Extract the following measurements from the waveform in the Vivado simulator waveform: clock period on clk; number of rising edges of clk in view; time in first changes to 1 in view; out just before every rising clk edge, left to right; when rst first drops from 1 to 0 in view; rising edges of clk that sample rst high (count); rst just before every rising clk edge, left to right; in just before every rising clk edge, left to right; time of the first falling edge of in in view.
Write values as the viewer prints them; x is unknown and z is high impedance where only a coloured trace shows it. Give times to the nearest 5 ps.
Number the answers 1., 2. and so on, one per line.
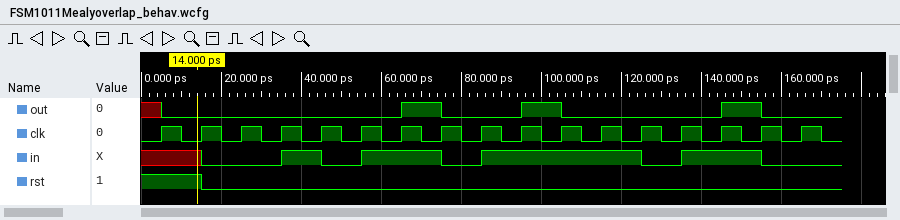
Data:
1. 10 ps
2. 17
3. 35 ps
4. x 0 0 0 0 0 0 1 0 0 1 0 0 0 0 1 0
5. 15 ps
6. 2
7. 1 1 0 0 0 0 0 0 0 0 0 0 0 0 0 0 0
8. x x 0 0 1 0 1 1 0 1 1 1 1 0 1 1 0
9. 45 ps
